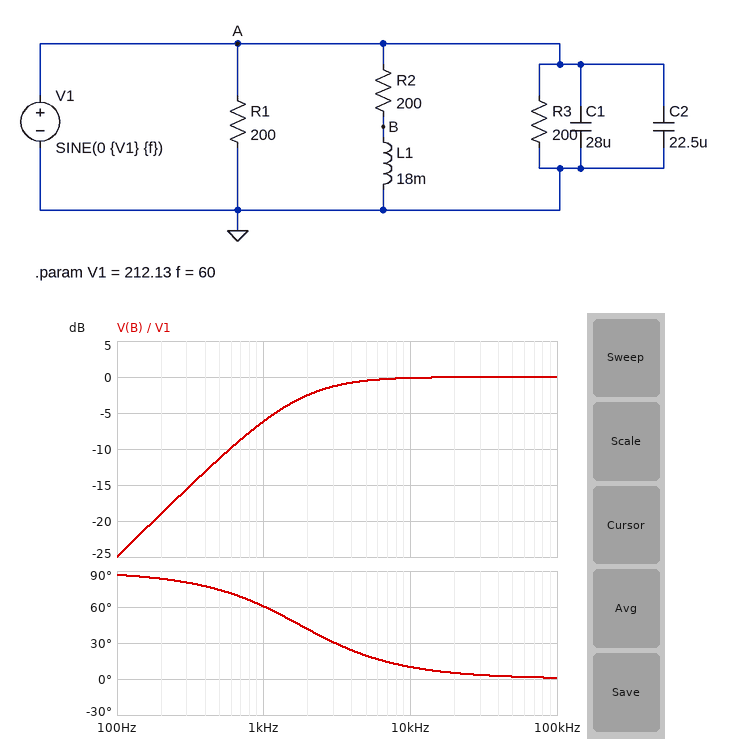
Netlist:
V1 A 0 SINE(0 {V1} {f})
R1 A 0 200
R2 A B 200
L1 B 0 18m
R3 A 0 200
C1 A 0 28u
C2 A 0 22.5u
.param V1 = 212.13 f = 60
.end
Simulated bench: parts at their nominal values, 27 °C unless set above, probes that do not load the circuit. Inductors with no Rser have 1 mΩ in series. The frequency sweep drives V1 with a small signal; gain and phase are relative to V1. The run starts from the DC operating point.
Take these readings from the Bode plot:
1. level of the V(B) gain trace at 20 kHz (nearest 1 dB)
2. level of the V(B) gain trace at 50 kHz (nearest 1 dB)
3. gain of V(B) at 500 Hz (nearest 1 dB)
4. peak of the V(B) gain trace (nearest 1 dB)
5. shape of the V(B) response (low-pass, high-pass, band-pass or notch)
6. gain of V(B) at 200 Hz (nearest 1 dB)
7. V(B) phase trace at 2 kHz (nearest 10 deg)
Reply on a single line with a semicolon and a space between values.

0 dB; 0 dB; -11 dB; 0 dB; high-pass; -19 dB; 40 deg
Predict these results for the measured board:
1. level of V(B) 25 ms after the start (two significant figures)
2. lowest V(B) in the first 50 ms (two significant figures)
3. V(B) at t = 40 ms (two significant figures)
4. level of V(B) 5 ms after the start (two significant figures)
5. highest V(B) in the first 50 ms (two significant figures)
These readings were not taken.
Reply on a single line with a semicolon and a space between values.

-7.2 V; -7.2 V; -5.7 V; -2.0 V; 7.2 V
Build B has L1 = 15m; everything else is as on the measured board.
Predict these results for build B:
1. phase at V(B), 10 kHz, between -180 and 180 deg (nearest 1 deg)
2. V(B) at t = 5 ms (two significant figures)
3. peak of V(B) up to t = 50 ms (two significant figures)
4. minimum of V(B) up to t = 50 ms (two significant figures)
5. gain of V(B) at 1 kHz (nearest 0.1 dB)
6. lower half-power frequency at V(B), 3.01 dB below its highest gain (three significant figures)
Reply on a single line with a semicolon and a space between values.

12 deg; -1.7 V; 6.0 V; -6.0 V; -7.4 dB; 2.12 kHz
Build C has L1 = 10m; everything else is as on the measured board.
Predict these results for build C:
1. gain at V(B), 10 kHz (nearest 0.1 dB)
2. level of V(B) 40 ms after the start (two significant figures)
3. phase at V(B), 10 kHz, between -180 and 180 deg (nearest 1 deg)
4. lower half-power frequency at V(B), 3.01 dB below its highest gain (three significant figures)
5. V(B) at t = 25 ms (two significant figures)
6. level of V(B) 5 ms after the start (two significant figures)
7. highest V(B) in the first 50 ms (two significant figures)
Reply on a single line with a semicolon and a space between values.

-0.4 dB; -3.2 V; 18 deg; 3.18 kHz; -4.0 V; -1.2 V; 4.0 V
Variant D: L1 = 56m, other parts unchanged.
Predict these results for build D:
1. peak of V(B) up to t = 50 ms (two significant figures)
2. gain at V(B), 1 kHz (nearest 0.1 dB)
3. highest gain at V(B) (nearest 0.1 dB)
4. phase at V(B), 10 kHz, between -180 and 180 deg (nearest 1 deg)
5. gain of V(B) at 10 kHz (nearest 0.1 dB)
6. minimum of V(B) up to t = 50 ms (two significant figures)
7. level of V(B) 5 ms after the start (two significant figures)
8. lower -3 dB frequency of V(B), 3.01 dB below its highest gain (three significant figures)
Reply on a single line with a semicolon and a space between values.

22 V; -1.2 dB; 0 dB; 3 deg; 0 dB; -22 V; -4.6 V; 568 Hz
